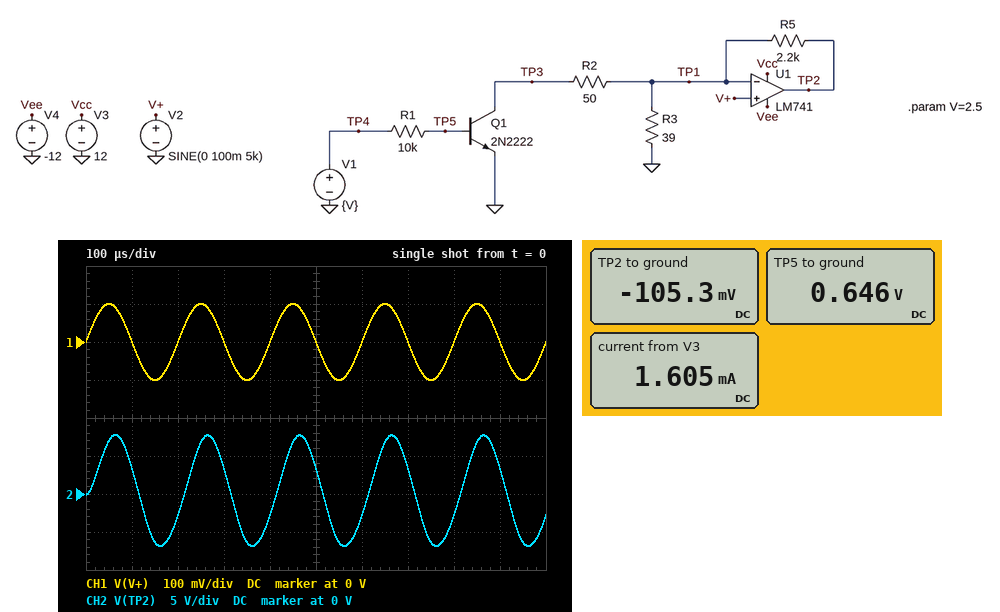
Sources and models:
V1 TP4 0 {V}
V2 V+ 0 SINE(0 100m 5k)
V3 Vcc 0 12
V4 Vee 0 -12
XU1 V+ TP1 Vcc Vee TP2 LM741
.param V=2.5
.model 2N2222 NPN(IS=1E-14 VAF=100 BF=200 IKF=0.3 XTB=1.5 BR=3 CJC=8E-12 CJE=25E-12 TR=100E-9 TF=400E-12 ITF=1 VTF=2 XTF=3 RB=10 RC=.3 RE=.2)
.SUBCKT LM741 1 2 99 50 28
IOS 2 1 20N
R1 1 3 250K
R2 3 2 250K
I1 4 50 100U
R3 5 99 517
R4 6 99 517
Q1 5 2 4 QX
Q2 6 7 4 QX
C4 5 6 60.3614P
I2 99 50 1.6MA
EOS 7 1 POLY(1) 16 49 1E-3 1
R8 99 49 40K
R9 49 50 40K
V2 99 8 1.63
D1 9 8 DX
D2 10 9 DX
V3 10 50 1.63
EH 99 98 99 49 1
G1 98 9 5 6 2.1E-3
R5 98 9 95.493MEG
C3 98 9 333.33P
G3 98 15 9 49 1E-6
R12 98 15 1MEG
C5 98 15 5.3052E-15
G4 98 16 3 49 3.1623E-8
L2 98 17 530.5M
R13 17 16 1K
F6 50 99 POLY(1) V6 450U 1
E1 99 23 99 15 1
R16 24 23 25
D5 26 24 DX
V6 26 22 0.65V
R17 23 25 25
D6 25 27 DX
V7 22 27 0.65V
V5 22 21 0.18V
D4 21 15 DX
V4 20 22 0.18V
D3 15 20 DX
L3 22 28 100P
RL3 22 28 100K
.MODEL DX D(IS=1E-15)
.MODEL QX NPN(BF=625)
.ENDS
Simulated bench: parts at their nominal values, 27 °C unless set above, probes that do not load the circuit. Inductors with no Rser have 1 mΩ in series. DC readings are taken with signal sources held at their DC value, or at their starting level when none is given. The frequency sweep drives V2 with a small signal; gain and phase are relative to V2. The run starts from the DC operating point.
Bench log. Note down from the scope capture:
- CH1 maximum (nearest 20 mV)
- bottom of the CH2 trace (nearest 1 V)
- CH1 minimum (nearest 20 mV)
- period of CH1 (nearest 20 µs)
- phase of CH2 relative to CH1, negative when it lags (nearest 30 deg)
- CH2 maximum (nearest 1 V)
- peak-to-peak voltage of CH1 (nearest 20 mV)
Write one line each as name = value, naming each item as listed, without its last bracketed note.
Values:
CH1 maximum = 100 mV
bottom of the CH2 trace = -7 V
CH1 minimum = -100 mV
period of CH1 = 200 µs
phase of CH2 relative to CH1, negative when it lags = -30 deg
CH2 maximum = 8 V
peak-to-peak voltage of CH1 = 200 mV
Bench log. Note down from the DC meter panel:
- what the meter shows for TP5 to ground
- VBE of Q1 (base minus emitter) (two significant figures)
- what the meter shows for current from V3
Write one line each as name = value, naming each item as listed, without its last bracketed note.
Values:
what the meter shows for TP5 to ground = 0.646 V
VBE of Q1 (base minus emitter) = 650 mV
what the meter shows for current from V3 = 1.605 mA
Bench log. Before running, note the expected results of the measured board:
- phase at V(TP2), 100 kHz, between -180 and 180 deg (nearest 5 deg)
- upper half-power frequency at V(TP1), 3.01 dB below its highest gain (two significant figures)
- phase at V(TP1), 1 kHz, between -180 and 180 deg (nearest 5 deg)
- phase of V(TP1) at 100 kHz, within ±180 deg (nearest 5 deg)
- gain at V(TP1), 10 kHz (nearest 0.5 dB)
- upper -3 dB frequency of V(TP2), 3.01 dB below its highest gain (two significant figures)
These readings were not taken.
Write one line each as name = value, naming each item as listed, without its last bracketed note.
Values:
phase at V(TP2), 100 kHz, between -180 and 180 deg = -85 deg
upper half-power frequency at V(TP1), 3.01 dB below its highest gain = 11 kHz
phase at V(TP1), 1 kHz, between -180 and 180 deg = -5 deg
phase of V(TP1) at 100 kHz, within ±180 deg = -85 deg
gain at V(TP1), 10 kHz = -2.5 dB
upper -3 dB frequency of V(TP2), 3.01 dB below its highest gain = 11 kHz
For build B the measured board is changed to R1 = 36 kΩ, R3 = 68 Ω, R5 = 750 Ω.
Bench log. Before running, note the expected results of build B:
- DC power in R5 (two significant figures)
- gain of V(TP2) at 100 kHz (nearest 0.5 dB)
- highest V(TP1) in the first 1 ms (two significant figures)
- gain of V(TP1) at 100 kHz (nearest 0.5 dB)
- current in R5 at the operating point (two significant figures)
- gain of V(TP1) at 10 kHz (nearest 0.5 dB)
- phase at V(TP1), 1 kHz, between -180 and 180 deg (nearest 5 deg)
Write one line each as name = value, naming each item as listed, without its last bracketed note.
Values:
DC power in R5 = 290 nW
gain of V(TP2) at 100 kHz = 17.5 dB
highest V(TP1) in the first 1 ms = 100 mV
gain of V(TP1) at 100 kHz = -6.5 dB
current in R5 at the operating point = 20 µA
gain of V(TP1) at 10 kHz = 0 dB
phase at V(TP1), 1 kHz, between -180 and 180 deg = 0 deg
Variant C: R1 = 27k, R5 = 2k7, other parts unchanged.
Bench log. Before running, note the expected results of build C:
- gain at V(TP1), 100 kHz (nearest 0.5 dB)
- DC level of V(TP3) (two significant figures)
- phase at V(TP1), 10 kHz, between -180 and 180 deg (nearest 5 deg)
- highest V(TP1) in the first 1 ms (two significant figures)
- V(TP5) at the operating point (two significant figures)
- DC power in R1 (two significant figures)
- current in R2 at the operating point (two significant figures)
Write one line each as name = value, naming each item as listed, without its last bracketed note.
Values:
gain at V(TP1), 100 kHz = -19.5 dB
DC level of V(TP3) = 3.1 mV
phase at V(TP1), 10 kHz, between -180 and 180 deg = -45 deg
highest V(TP1) in the first 1 ms = 89 mV
V(TP5) at the operating point = 620 mV
DC power in R1 = 130 µW
current in R2 at the operating point = 42 µA
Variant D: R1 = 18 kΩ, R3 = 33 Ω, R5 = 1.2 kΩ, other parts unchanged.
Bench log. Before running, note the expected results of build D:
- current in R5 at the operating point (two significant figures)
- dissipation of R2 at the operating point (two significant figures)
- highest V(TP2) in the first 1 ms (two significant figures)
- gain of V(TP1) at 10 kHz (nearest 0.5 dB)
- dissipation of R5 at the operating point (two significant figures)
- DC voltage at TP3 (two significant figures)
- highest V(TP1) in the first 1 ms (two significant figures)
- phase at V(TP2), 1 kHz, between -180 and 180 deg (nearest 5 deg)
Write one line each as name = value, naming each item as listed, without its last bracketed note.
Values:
current in R5 at the operating point = 24 µA
dissipation of R2 at the operating point = 150 nW
highest V(TP2) in the first 1 ms = 4.9 V
gain of V(TP1) at 10 kHz = -1.0 dB
dissipation of R5 at the operating point = 710 nW
DC voltage at TP3 = 3.7 mV
highest V(TP1) in the first 1 ms = 97 mV
phase at V(TP2), 1 kHz, between -180 and 180 deg = -5 deg
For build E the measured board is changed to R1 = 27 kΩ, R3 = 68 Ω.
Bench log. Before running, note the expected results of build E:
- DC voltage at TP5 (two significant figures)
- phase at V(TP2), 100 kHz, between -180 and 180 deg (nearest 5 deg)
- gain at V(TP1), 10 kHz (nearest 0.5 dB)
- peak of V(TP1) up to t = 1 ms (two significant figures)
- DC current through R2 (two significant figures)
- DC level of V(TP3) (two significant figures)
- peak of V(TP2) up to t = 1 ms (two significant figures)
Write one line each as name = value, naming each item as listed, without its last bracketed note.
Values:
DC voltage at TP5 = 620 mV
phase at V(TP2), 100 kHz, between -180 and 180 deg = -80 deg
gain at V(TP1), 10 kHz = -1.0 dB
peak of V(TP1) up to t = 1 ms = 96 mV
DC current through R2 = 42 µA
DC level of V(TP3) = 3.1 mV
peak of V(TP2) up to t = 1 ms = 5.3 V
